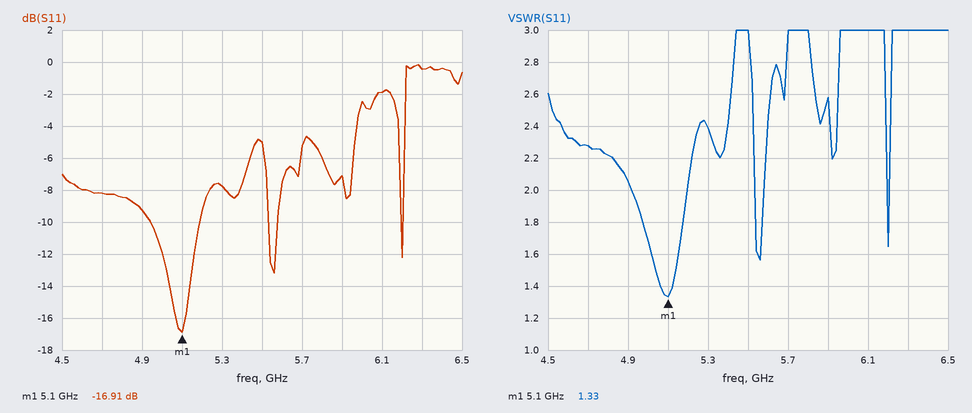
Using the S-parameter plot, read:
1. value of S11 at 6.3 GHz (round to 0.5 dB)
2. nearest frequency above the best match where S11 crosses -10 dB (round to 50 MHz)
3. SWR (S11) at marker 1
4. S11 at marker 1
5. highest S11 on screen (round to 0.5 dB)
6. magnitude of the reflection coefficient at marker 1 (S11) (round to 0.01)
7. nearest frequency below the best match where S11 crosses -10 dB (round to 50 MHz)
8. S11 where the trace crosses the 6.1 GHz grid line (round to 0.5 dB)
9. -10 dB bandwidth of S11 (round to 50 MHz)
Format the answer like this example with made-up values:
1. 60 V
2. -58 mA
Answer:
1. -0.5 dB
2. 5.20 GHz
3. 1.33
4. -16.91 dB
5. 0.0 dB
6. 0.14
7. 4.95 GHz
8. -2.0 dB
9. 250 MHz
